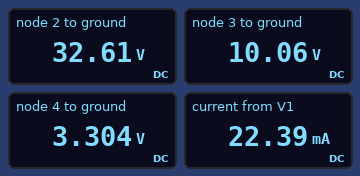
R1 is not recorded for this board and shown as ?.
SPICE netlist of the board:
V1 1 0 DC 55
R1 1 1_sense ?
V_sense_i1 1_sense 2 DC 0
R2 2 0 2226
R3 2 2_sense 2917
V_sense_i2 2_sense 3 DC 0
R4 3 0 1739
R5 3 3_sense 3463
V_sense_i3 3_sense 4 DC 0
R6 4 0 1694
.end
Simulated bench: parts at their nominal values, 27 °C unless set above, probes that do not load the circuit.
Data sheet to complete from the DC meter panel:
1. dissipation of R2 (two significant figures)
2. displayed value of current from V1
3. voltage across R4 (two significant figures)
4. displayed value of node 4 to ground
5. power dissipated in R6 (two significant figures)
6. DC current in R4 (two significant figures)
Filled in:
480 mW
22.39 mA
10 V
3.304 V
6.4 mW
5.8 mA
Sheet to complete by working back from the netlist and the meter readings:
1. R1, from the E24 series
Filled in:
1 kΩ
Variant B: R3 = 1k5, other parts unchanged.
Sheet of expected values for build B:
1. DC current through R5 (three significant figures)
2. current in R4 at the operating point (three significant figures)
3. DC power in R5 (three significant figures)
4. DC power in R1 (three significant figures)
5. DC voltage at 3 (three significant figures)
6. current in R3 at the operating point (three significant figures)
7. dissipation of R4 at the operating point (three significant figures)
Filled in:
2.74 mA
8.13 mA
26.0 mW
603 mW
14.1 V
10.9 mA
115 mW
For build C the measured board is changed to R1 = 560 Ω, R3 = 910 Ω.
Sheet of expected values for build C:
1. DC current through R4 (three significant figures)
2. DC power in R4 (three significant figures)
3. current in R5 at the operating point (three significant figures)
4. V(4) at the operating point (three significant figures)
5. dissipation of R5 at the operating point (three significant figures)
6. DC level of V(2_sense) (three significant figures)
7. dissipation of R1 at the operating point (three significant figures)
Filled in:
12.4 mA
266 mW
4.17 mA
7.06 V
60.2 mW
21.5 V
608 mW
